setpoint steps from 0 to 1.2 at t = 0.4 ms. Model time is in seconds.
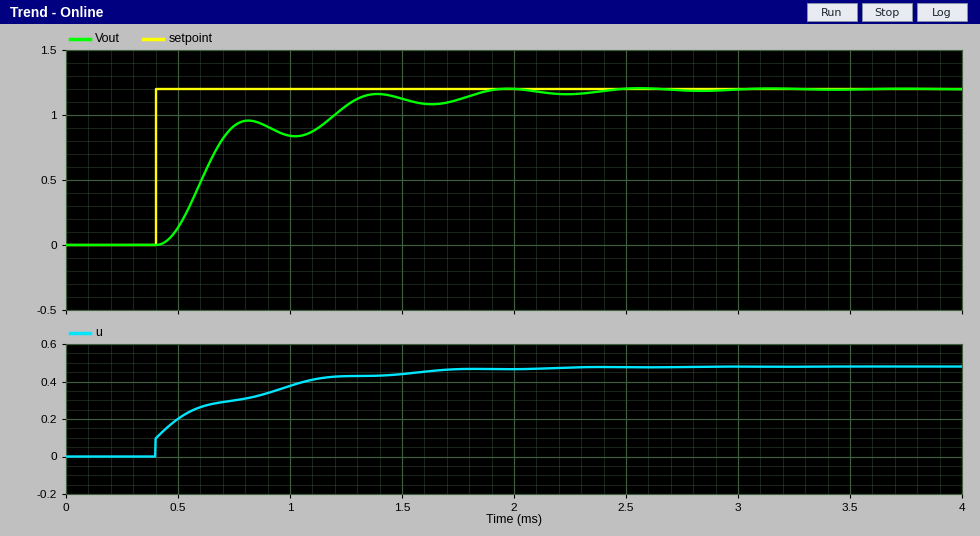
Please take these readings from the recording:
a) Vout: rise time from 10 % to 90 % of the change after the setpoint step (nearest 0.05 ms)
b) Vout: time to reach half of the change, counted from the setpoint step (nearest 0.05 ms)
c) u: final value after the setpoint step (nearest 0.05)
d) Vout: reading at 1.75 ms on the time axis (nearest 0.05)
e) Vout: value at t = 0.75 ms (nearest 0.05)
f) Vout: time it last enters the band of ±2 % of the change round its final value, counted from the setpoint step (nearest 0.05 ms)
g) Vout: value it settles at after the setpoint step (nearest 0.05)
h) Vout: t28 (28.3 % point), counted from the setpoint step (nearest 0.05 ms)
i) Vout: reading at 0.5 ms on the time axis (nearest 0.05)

0.75 ms
0.25 ms
0.50
1.10
0.90
1.95 ms
1.20
0.15 ms
0.15
